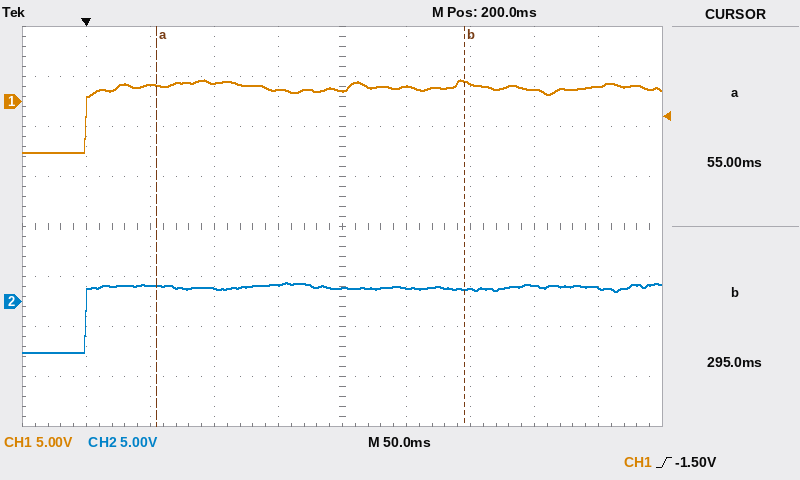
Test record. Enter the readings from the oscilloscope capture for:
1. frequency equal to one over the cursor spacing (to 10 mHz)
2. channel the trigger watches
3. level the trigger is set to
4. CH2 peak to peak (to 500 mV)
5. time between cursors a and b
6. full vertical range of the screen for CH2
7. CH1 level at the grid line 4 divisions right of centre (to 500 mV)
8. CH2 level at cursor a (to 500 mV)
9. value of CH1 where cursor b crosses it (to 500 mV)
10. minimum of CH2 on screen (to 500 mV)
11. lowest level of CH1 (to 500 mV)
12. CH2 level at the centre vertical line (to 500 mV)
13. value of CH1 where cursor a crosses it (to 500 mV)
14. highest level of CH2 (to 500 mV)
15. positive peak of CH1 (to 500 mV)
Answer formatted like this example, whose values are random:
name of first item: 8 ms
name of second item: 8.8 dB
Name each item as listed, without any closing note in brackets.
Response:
frequency equal to one over the cursor spacing: 4.17 Hz
channel the trigger watches: CH1
level the trigger is set to: -1.50 V
CH2 peak to peak: 7.0 V
time between cursors a and b: 240 ms
full vertical range of the screen for CH2: 40 V
CH1 level at the grid line 4 divisions right of centre: 1.5 V
CH2 level at cursor a: 1.5 V
value of CH1 where cursor b crosses it: 2.0 V
minimum of CH2 on screen: -5.0 V
lowest level of CH1: -5.0 V
CH2 level at the centre vertical line: 1.5 V
value of CH1 where cursor a crosses it: 1.5 V
highest level of CH2: 2.0 V
positive peak of CH1: 2.0 V
